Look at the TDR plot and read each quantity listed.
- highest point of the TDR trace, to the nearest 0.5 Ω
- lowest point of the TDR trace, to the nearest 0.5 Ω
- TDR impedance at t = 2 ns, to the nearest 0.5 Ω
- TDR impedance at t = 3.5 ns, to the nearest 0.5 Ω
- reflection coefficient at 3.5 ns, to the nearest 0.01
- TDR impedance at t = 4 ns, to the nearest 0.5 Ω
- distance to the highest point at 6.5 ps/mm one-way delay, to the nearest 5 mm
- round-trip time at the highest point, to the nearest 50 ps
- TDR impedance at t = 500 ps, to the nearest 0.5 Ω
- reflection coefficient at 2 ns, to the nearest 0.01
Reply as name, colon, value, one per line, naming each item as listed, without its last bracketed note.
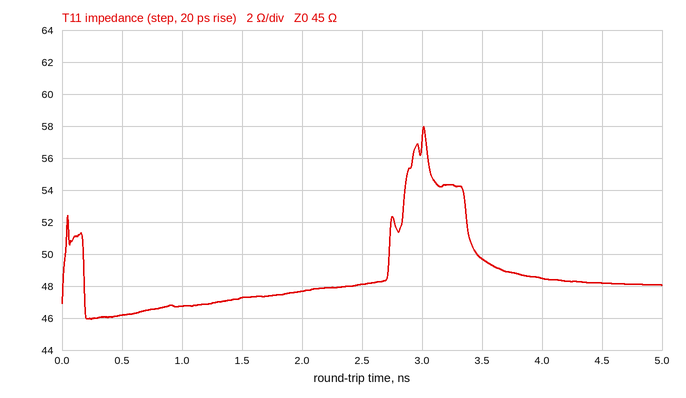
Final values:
highest point of the TDR trace, to the nearest 0.5 Ω: 58.0 Ω
lowest point of the TDR trace, to the nearest 0.5 Ω: 46.0 Ω
TDR impedance at t = 2 ns, to the nearest 0.5 Ω: 47.5 Ω
TDR impedance at t = 3.5 ns, to the nearest 0.5 Ω: 49.5 Ω
reflection coefficient at 3.5 ns, to the nearest 0.01: +0.05
TDR impedance at t = 4 ns, to the nearest 0.5 Ω: 48.5 Ω
distance to the highest point at 6.5 ps/mm one-way delay, to the nearest 5 mm: 230 mm
round-trip time at the highest point, to the nearest 50 ps: 3.00 ns
TDR impedance at t = 500 ps, to the nearest 0.5 Ω: 46.0 Ω
reflection coefficient at 2 ns, to the nearest 0.01: +0.03
